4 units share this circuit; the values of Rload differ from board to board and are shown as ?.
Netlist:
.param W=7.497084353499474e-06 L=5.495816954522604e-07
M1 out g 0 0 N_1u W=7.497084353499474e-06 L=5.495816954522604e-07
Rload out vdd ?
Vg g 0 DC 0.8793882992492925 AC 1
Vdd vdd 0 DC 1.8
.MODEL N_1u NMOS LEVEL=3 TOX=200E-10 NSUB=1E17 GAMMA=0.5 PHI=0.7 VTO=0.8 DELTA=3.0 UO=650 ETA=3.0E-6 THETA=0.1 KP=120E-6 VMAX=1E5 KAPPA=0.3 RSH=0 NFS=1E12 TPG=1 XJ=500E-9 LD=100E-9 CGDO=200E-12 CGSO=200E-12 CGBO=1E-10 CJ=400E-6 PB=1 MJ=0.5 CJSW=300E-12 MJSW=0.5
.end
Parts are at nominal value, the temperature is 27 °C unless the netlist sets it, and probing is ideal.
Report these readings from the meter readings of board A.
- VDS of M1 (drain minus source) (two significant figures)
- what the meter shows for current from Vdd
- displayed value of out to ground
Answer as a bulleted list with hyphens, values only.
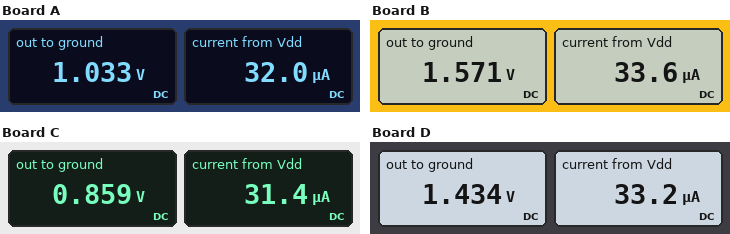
- 1.0 V
- 32.0 µA
- 1.033 V
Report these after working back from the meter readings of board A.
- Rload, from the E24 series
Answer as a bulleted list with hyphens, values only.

- 24 kΩ
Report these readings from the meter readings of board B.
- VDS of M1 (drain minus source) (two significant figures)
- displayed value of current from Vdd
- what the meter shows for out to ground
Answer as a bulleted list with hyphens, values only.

- 1.6 V
- 33.6 µA
- 1.571 V
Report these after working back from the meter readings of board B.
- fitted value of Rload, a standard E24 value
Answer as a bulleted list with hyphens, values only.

- 6.8 kΩ
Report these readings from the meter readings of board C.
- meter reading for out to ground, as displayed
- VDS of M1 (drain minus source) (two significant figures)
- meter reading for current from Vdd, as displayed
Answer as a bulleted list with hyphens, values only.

- 0.859 V
- 860 mV
- 31.4 µA
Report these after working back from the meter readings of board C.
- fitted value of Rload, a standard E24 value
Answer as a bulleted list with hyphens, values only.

- 30 kΩ
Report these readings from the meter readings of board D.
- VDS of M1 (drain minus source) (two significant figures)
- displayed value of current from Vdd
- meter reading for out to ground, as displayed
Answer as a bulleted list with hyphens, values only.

- 1.4 V
- 33.2 µA
- 1.434 V
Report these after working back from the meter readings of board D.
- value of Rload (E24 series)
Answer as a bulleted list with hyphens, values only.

- 11 kΩ
